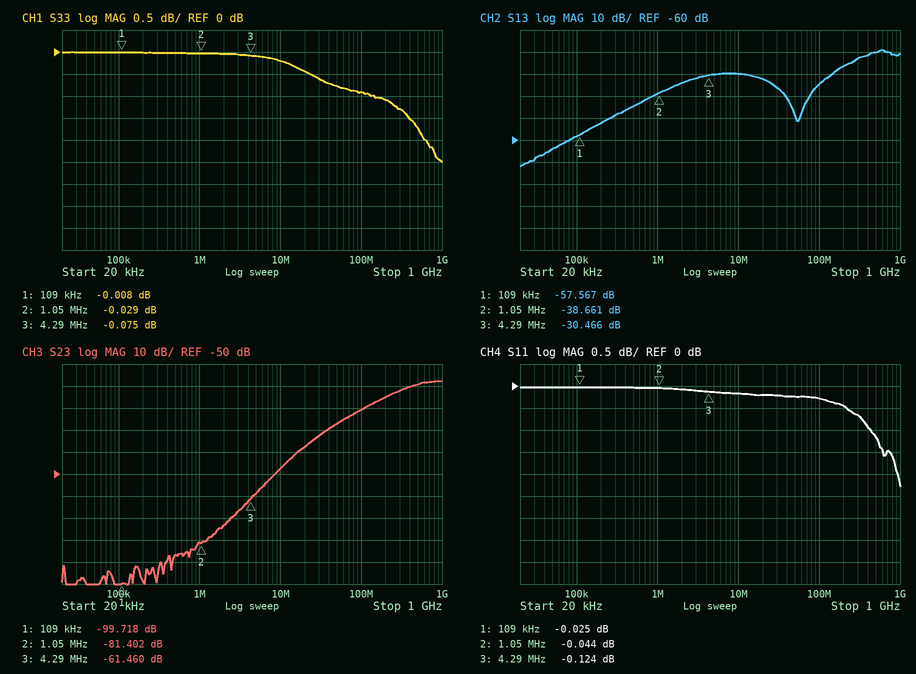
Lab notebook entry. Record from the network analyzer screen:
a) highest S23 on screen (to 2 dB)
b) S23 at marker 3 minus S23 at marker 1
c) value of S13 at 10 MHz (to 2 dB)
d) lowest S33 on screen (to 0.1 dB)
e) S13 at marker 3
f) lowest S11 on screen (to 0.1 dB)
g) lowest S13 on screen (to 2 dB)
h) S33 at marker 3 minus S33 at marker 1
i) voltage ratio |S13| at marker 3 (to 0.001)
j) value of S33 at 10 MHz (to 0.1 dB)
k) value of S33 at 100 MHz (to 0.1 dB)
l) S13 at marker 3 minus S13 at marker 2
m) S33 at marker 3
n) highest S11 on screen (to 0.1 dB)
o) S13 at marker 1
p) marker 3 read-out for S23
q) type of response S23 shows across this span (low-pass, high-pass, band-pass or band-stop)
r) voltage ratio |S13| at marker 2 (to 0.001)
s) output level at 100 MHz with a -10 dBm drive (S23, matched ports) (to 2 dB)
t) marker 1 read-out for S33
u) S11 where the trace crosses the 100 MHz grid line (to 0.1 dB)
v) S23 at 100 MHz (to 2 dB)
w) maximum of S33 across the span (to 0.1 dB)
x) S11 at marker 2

-8 dB
38.258 dB
-30 dB
-2.5 dB
-30.466 dB
-2.3 dB
-72 dB
-0.067 dB
0.030
-0.2 dB
-0.9 dB
8.195 dB
-0.075 dB
0.0 dB
-57.567 dB
-61.460 dB
high-pass
0.012
-30 dBm
-0.008 dB
-0.3 dB
-20 dB
0.0 dB
-0.044 dB
